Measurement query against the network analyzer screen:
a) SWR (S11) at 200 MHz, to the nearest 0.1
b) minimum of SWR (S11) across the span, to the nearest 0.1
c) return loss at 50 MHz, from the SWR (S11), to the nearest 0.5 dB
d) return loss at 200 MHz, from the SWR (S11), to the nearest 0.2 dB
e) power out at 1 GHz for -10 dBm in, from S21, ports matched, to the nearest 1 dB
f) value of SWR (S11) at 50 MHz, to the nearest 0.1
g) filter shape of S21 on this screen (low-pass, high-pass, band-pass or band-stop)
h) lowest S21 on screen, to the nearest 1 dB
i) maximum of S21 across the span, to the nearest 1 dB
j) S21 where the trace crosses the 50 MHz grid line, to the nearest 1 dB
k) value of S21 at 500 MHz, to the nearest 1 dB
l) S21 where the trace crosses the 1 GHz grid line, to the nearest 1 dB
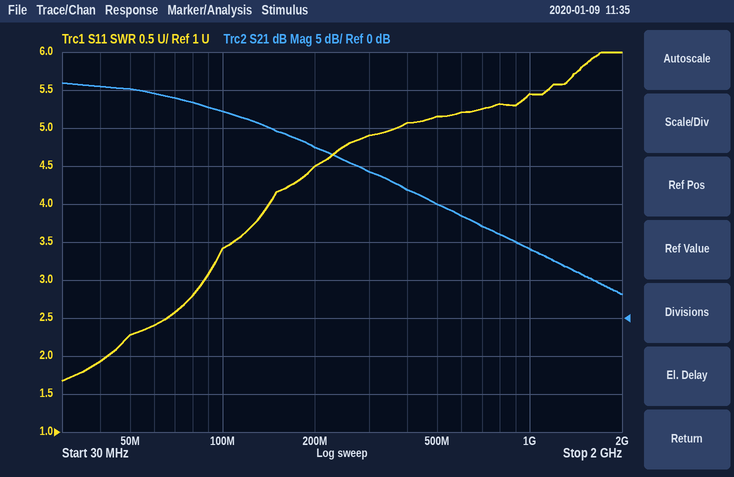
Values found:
4.5
1.7
8.0 dB
4.0 dB
-1 dBm
2.3
low-pass
3 dB
31 dB
30 dB
15 dB
9 dB
